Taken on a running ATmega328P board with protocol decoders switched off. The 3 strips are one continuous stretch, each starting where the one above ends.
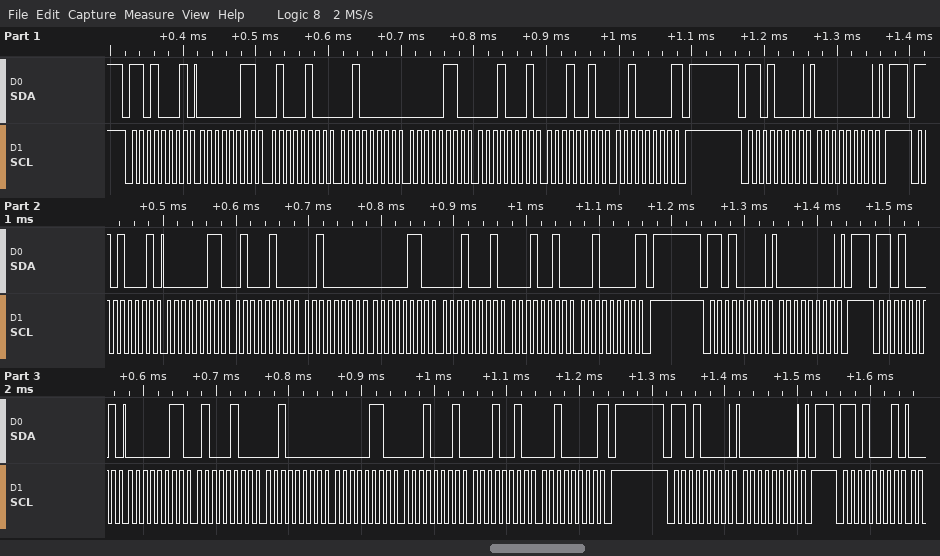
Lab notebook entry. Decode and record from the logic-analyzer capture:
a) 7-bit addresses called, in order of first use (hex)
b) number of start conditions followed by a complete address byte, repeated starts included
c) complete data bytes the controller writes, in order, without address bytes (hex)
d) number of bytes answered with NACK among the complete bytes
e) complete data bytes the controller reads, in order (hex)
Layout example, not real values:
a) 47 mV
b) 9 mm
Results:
a) 0x68
b) 7
c) 00 00 00
d) 3
e) 03 44 20 06 11 12 20 03 44 20 06 11 12 20 03 44 20 06 11 12 20
